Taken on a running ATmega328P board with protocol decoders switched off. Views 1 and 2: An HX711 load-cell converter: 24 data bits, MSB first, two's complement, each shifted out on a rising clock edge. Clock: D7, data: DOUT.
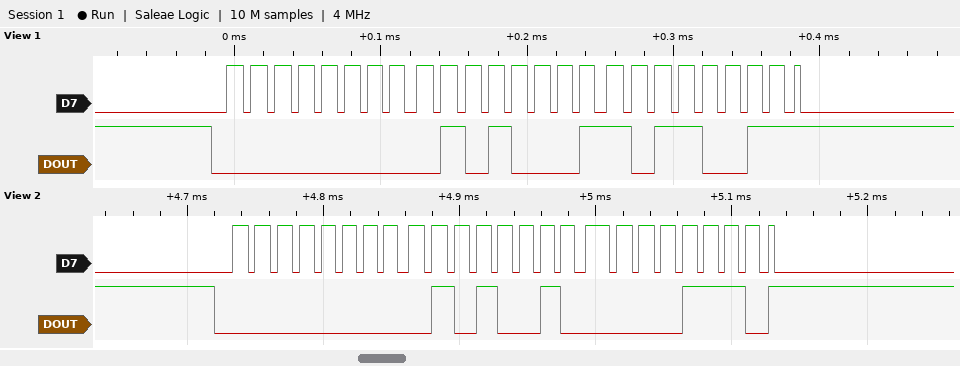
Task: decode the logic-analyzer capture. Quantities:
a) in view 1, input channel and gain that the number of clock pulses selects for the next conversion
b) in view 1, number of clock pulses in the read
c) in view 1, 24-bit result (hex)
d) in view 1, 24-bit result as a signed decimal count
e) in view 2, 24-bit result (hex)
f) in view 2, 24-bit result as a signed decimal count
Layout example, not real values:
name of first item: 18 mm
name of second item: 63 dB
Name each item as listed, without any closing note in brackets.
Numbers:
in view 1, input channel and gain that the number of clock pulses selects for the next conversion: channel A, gain 128
in view 1, number of clock pulses in the read: 25
in view 1, 24-bit result: 0x0051B3
in view 1, 24-bit result as a signed decimal count: 20915
in view 2, 24-bit result: 0x00520E
in view 2, 24-bit result as a signed decimal count: 21006
